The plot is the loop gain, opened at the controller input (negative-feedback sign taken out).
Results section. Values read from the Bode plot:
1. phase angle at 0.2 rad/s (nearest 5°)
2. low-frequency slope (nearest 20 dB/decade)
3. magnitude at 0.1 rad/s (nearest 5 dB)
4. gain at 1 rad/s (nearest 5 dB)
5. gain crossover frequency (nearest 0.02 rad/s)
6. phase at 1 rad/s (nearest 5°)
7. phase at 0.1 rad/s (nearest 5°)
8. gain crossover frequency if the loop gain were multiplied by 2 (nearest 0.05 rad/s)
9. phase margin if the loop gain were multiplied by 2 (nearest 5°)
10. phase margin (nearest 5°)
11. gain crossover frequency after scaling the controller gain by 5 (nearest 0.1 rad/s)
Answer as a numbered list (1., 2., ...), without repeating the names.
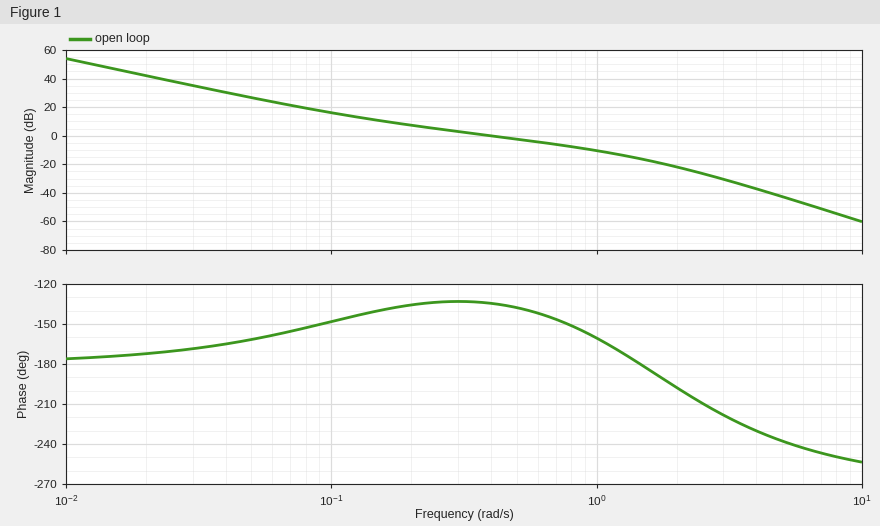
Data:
1. -135°
2. -40 dB/decade
3. 15 dB
4. -10 dB
5. 0.40 rad/s
6. -160°
7. -150°
8. 0.70 rad/s
9. 35°
10. 45°
11. 1.3 rad/s
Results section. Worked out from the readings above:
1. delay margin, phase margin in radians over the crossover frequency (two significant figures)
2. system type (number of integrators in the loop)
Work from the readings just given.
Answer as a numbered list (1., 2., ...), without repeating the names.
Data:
1. 2.0 s
2. 2
